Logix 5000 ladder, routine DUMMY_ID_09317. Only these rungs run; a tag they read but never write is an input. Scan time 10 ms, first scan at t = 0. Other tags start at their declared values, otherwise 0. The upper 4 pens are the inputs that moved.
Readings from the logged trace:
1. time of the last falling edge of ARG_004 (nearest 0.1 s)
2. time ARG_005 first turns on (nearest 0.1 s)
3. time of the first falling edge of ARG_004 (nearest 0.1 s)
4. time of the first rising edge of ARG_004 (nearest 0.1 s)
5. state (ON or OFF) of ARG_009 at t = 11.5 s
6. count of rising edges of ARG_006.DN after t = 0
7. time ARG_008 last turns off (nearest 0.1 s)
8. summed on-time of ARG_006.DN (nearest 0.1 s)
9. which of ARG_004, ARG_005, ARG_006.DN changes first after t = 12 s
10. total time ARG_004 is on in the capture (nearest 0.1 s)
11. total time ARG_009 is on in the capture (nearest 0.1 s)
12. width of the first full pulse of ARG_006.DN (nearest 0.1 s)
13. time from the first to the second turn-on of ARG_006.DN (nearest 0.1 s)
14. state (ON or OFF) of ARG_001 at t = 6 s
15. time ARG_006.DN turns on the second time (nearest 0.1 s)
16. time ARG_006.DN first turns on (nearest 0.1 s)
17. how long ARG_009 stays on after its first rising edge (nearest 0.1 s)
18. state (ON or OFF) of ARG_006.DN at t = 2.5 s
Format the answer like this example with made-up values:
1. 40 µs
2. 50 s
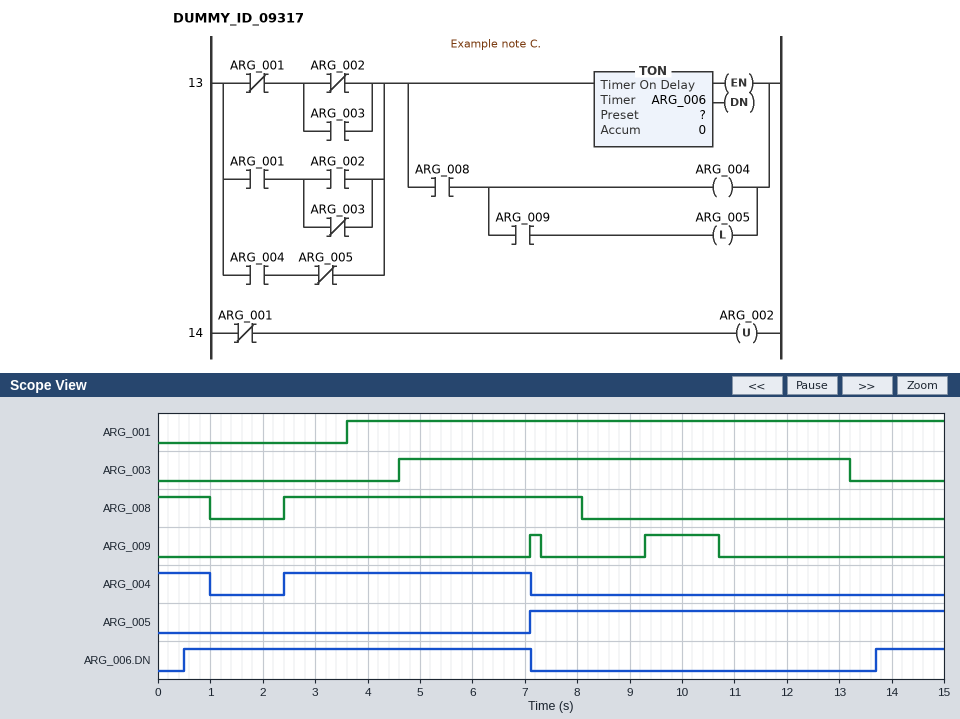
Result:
1. 7.1 s
2. 7.1 s
3. 1.0 s
4. 2.4 s
5. OFF
6. 2
7. 8.1 s
8. 7.9 s
9. ARG_006.DN
10. 5.7 s
11. 1.6 s
12. 6.6 s
13. 13.2 s
14. ON
15. 13.7 s
16. 0.5 s
17. 0.2 s
18. ON
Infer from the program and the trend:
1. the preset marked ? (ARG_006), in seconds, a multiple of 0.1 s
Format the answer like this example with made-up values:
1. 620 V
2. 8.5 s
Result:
1. 0.5 s
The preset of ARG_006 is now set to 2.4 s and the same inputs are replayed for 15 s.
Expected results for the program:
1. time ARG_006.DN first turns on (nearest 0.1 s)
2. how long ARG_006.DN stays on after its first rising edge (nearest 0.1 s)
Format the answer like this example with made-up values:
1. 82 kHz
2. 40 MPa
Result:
1. 2.4 s
2. 4.7 s
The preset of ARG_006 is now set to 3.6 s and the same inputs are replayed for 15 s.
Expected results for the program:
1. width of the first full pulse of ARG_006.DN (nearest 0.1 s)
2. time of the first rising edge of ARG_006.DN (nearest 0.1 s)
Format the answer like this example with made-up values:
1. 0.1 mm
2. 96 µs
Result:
1. 3.5 s
2. 3.6 s
